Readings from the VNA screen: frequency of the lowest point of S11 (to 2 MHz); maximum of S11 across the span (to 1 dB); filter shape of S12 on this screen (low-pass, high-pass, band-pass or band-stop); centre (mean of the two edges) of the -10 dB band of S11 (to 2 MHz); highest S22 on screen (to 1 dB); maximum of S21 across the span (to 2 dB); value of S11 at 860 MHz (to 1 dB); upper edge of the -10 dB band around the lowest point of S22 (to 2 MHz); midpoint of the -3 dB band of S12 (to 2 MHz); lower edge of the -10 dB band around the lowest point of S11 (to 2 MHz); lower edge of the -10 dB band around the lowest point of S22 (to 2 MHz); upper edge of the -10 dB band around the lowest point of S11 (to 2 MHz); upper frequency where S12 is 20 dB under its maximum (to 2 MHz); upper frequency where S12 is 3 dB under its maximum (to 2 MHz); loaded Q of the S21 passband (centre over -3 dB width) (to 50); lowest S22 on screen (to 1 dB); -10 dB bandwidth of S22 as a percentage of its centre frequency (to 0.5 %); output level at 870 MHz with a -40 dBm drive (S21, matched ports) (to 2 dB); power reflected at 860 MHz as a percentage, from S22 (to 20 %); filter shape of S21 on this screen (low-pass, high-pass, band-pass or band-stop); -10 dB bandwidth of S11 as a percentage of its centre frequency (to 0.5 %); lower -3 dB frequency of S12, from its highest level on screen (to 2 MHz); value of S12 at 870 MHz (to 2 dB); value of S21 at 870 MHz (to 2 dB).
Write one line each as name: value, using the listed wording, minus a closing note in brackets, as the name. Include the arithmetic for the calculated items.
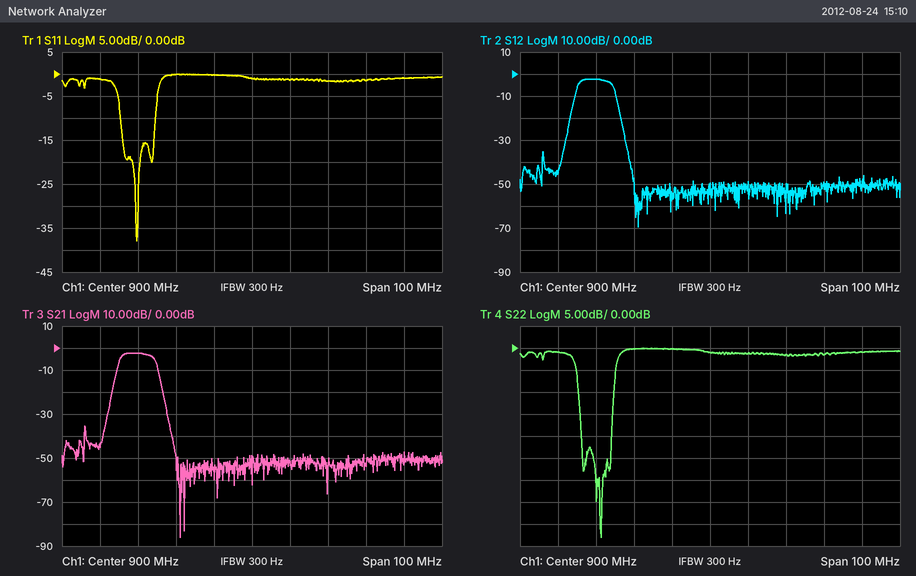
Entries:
frequency of the lowest point of S11: 870 MHz
maximum of S11 across the span: 0 dB
filter shape of S12 on this screen: band-pass
centre (mean of the two edges) of the -10 dB band of S11: 870 MHz
highest S22 on screen: 0 dB
maximum of S21 across the span: -2 dB
value of S11 at 860 MHz: -1 dB
upper edge of the -10 dB band around the lowest point of S22: 874 MHz
midpoint of the -3 dB band of S12: 870 MHz
lower edge of the -10 dB band around the lowest point of S11: 866 MHz
lower edge of the -10 dB band around the lowest point of S22: 866 MHz
upper edge of the -10 dB band around the lowest point of S11: 874 MHz
upper frequency where S12 is 20 dB under its maximum: 876 MHz
upper frequency where S12 is 3 dB under its maximum: 874 MHz
loaded Q of the S21 passband (centre over -3 dB width): 870 MHz / 8 MHz ≈ 109, so 100 to the nearest 50
lowest S22 on screen: -43 dB
-10 dB bandwidth of S22 as a percentage of its centre frequency: 8 MHz / 870 MHz ≈ 0.920 %, so 1.0 % to the nearest 0.5 %
output level at 870 MHz with a -40 dBm drive (S21, matched ports): -40 dBm + (-2 dB) = -42 dBm
power reflected at 860 MHz as a percentage, from S22: 10^(-1/10) ≈ 79.4 %, so 80 % to the nearest 20 %
filter shape of S21 on this screen: band-pass
-10 dB bandwidth of S11 as a percentage of its centre frequency: 8 MHz / 870 MHz ≈ 0.920 %, so 1.0 % to the nearest 0.5 %
lower -3 dB frequency of S12, from its highest level on screen: 866 MHz
value of S12 at 870 MHz: -2 dB
value of S21 at 870 MHz: -2 dB
